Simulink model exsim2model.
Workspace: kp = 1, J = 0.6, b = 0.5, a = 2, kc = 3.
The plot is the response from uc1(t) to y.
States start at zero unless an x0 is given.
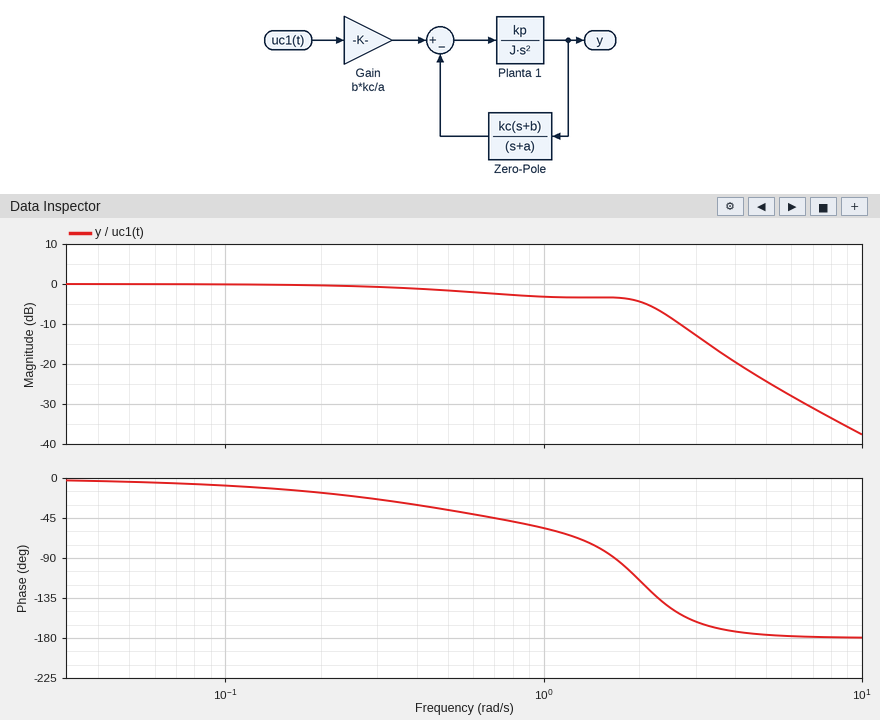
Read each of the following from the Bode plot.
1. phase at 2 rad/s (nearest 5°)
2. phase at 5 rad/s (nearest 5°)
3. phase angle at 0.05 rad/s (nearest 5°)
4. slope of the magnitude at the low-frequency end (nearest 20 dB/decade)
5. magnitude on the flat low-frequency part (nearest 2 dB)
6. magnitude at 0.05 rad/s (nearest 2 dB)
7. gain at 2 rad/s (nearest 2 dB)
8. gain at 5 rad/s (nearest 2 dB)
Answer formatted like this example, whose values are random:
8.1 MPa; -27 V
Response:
-115°; -175°; -5°; 0 dB/decade; 0 dB; 0 dB; -4 dB; -24 dB
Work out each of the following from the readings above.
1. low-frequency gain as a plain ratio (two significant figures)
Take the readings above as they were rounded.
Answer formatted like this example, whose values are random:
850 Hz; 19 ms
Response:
1.0
